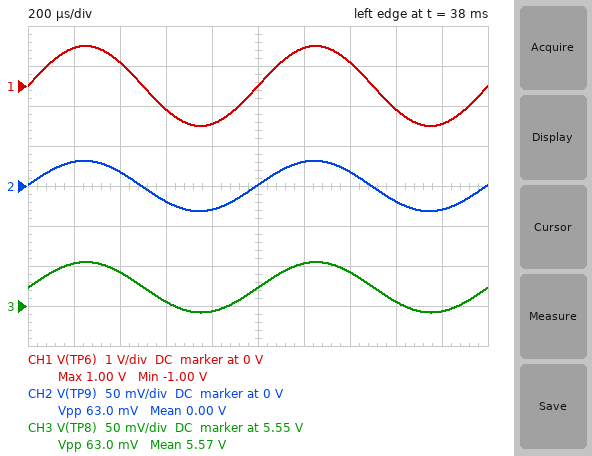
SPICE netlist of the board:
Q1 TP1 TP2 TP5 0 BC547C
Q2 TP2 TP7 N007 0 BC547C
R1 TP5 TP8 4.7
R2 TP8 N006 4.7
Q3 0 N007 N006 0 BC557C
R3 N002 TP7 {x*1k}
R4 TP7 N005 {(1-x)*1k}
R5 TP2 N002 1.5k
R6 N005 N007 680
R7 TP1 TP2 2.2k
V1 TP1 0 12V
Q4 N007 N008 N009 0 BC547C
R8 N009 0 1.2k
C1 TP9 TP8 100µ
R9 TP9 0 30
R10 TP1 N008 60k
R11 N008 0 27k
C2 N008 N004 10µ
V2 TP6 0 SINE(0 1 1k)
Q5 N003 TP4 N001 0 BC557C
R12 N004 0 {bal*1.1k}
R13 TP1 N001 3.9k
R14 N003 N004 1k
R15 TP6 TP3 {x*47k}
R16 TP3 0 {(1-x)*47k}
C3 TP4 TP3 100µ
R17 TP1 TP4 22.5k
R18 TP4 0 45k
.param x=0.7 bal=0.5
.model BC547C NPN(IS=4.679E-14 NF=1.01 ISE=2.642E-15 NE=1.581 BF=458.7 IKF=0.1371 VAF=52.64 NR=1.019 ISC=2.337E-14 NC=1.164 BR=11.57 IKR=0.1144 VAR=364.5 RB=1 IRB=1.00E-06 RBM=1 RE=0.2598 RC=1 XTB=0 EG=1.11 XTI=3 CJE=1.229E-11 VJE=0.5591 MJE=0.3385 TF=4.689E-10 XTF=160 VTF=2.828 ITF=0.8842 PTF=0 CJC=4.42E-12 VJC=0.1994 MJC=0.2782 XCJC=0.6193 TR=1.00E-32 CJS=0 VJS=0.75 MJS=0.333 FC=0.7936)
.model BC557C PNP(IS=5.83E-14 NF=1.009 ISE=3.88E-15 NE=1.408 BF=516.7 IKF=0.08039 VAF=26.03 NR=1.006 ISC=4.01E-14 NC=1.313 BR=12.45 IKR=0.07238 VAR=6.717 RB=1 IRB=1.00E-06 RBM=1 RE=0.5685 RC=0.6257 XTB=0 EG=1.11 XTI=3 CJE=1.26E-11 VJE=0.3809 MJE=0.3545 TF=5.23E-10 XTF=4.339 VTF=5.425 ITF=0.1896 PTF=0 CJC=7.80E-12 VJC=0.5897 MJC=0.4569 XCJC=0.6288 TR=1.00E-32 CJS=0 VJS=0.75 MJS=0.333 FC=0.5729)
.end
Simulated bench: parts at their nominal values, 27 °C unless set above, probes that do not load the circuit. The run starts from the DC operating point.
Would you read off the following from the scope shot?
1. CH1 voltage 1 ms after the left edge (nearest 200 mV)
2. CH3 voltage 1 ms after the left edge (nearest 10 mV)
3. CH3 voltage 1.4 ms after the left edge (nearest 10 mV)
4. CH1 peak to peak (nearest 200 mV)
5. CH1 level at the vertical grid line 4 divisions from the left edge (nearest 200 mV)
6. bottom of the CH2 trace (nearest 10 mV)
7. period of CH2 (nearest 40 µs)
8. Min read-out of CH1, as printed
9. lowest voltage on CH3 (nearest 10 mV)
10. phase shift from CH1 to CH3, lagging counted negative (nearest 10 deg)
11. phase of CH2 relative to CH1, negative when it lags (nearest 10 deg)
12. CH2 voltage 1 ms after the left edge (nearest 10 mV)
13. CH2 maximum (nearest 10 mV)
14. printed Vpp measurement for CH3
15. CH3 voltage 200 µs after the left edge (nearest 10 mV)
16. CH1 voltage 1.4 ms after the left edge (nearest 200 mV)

0 V
5.57 V
5.59 V
2.0 V
-1.0 V
-30 mV
1.00 ms
-1.00 V
5.54 V
0 deg
0 deg
0 V
30 mV
63.0 mV
5.60 V
600 mV
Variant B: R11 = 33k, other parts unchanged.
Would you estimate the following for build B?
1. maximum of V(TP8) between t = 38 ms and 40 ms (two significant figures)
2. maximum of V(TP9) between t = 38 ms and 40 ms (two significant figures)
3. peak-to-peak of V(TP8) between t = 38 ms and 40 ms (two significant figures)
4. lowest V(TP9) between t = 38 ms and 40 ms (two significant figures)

4.7 V
30 mV
58 mV
-28 mV
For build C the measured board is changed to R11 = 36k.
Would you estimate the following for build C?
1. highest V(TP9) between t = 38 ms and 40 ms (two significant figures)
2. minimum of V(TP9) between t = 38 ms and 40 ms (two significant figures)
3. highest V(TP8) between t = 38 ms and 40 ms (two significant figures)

14 mV
-8.3 mV
4.7 V
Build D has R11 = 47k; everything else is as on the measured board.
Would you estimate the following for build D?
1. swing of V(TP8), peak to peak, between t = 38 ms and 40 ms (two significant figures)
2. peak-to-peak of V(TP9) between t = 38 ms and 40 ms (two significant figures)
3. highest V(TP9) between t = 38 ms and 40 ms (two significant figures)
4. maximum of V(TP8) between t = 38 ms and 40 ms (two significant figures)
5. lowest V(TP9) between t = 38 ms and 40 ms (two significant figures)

7.1 mV
7.2 mV
4.4 mV
4.7 V
-2.8 mV
